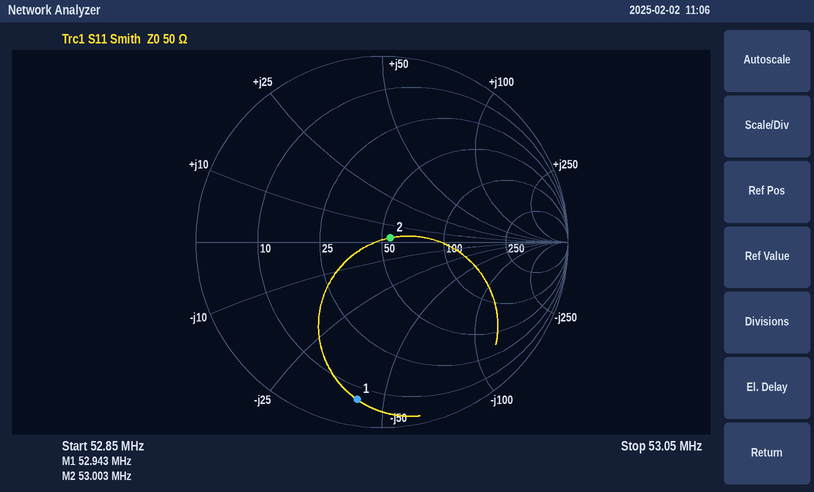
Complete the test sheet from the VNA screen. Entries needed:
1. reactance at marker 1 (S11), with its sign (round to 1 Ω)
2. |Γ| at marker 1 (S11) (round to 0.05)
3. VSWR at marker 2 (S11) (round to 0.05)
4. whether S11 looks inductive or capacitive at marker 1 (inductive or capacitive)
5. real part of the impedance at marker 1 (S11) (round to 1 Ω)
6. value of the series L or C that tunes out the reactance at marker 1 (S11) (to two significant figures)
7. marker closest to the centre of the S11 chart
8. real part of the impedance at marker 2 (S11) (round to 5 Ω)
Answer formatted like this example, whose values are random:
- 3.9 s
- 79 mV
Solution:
- -42 Ω
- 0.85
- 1.10
- capacitive
- 7 Ω
- 130 nH
- marker 2
- 55 Ω
